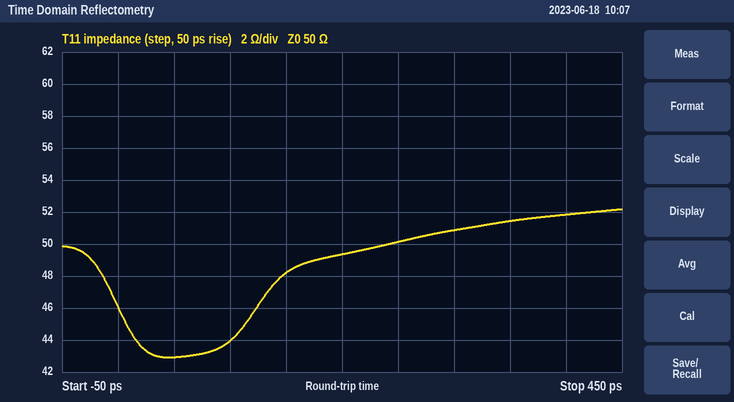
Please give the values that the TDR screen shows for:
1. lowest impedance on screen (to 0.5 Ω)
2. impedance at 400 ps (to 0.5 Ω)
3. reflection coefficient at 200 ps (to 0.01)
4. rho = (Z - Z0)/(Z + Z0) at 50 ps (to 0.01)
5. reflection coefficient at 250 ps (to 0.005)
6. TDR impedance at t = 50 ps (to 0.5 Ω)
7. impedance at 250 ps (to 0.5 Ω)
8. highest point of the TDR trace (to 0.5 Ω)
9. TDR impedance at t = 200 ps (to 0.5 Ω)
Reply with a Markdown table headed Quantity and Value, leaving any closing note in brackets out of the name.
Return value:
| Quantity | Value |
|---|---|
| lowest impedance on screen | 43.0 Ω |
| impedance at 400 ps | 52.0 Ω |
| reflection coefficient at 200 ps | -0.01 |
| rho = (Z - Z0)/(Z + Z0) at 50 ps | -0.08 |
| reflection coefficient at 250 ps | 0.000 |
| TDR impedance at t = 50 ps | 43.0 Ω |
| impedance at 250 ps | 50.0 Ω |
| highest point of the TDR trace | 52.0 Ω |
| TDR impedance at t = 200 ps | 49.5 Ω |
